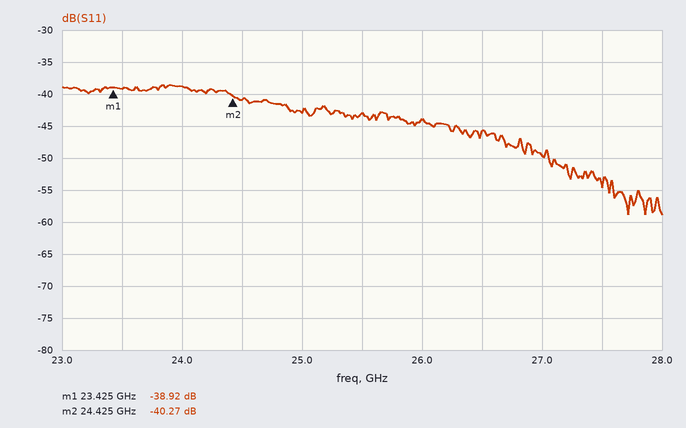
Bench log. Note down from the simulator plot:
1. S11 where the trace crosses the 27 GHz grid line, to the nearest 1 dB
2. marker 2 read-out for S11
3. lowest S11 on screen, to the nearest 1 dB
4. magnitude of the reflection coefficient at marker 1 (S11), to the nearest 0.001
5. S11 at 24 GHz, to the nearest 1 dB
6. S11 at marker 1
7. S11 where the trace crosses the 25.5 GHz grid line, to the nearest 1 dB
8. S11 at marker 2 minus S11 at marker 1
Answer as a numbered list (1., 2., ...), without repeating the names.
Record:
1. -50 dB
2. -40.27 dB
3. -59 dB
4. 0.011
5. -39 dB
6. -38.92 dB
7. -43 dB
8. -1.35 dB
